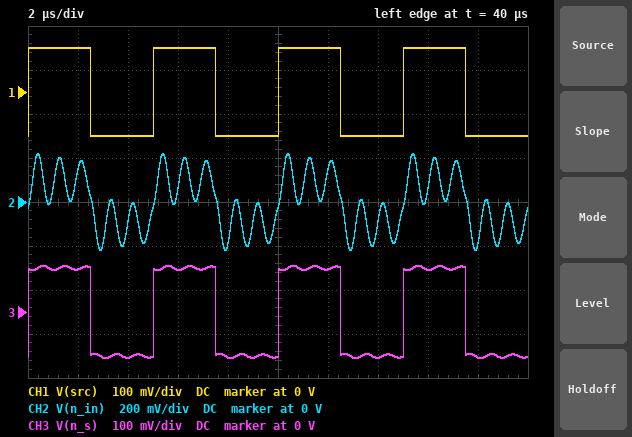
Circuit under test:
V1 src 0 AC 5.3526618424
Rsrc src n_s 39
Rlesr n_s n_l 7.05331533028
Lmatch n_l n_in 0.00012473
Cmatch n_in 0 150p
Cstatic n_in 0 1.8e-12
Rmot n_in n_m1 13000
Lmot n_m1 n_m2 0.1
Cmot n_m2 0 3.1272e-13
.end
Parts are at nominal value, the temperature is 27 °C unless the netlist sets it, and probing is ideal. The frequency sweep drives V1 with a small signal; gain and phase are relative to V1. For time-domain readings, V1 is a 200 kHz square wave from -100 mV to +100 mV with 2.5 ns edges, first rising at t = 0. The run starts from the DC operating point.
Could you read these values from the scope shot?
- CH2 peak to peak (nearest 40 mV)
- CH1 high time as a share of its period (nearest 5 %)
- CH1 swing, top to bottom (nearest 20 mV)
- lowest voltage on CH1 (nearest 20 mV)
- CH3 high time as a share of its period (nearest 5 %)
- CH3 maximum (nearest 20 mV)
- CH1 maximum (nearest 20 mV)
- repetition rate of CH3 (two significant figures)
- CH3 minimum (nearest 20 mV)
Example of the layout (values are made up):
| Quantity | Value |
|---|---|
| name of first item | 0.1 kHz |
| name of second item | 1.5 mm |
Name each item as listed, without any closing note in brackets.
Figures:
| Quantity | Value |
|---|---|
| CH2 peak to peak | 440 mV |
| CH1 high time as a share of its period | 50 % |
| CH1 swing, top to bottom | 200 mV |
| lowest voltage on CH1 | -100 mV |
| CH3 high time as a share of its period | 50 % |
| CH3 maximum | 100 mV |
| CH1 maximum | 100 mV |
| repetition rate of CH3 | 200 kHz |
| CH3 minimum | -100 mV |
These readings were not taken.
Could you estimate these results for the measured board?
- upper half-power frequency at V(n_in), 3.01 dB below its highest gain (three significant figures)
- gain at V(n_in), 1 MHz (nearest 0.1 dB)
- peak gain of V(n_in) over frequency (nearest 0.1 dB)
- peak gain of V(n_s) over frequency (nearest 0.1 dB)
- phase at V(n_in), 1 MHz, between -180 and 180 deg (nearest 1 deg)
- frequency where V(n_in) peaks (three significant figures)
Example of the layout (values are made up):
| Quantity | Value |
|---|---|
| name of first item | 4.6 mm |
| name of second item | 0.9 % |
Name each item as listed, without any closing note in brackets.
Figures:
| Quantity | Value |
|---|---|
| upper half-power frequency at V(n_in), 3.01 dB below its highest gain | 1.19 MHz |
| gain at V(n_in), 1 MHz | 11.6 dB |
| peak gain of V(n_in) over frequency | 25.9 dB |
| peak gain of V(n_s) over frequency | 0 dB |
| phase at V(n_in), 1 MHz, between -180 and 180 deg | -10 deg |
| frequency where V(n_in) peaks | 1.16 MHz |
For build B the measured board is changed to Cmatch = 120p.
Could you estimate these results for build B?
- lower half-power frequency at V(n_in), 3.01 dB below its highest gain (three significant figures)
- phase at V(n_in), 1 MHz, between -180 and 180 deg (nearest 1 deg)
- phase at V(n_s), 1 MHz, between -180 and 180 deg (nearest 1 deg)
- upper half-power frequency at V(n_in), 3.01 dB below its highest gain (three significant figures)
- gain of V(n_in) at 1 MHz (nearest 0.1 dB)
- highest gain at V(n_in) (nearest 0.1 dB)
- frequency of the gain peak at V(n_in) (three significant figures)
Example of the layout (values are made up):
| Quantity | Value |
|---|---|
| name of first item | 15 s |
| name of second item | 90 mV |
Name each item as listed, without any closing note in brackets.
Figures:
| Quantity | Value |
|---|---|
| lower half-power frequency at V(n_in), 3.01 dB below its highest gain | 1.26 MHz |
| phase at V(n_in), 1 MHz, between -180 and 180 deg | -5 deg |
| phase at V(n_s), 1 MHz, between -180 and 180 deg | -4 deg |
| upper half-power frequency at V(n_in), 3.01 dB below its highest gain | 1.32 MHz |
| gain of V(n_in) at 1 MHz | 7.8 dB |
| highest gain at V(n_in) | 26.8 dB |
| frequency of the gain peak at V(n_in) | 1.29 MHz |
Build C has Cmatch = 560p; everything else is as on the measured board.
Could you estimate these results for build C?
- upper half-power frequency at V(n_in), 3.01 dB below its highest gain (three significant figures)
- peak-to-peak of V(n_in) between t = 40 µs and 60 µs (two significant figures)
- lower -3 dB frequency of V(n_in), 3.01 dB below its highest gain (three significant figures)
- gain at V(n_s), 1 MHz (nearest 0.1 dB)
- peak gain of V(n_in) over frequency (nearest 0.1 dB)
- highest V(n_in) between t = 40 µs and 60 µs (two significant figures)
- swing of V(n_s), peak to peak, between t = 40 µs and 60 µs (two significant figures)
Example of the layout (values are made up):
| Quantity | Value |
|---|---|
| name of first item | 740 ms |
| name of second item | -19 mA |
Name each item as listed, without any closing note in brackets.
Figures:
| Quantity | Value |
|---|---|
| upper half-power frequency at V(n_in), 3.01 dB below its highest gain | 628 kHz |
| peak-to-peak of V(n_in) between t = 40 µs and 60 µs | 1.1 V |
| lower -3 dB frequency of V(n_in), 3.01 dB below its highest gain | 569 kHz |
| gain at V(n_s), 1 MHz | 0 dB |
| peak gain of V(n_in) over frequency | 20.2 dB |
| highest V(n_in) between t = 40 µs and 60 µs | 560 mV |
| swing of V(n_s), peak to peak, between t = 40 µs and 60 µs | 270 mV |
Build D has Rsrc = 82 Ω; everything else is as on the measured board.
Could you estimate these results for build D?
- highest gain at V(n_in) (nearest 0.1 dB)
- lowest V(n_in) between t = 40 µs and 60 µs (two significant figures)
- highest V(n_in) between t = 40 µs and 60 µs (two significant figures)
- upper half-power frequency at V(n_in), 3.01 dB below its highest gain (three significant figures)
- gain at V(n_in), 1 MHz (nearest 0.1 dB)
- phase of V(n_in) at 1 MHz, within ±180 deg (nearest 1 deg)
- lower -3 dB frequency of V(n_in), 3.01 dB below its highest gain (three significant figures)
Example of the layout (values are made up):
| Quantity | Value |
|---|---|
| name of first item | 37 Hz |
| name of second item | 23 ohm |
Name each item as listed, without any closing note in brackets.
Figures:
| Quantity | Value |
|---|---|
| highest gain at V(n_in) | 20.2 dB |
| lowest V(n_in) between t = 40 µs and 60 µs | -230 mV |
| highest V(n_in) between t = 40 µs and 60 µs | 230 mV |
| upper half-power frequency at V(n_in), 3.01 dB below its highest gain | 1.21 MHz |
| gain at V(n_in), 1 MHz | 11.3 dB |
| phase of V(n_in) at 1 MHz, within ±180 deg | -18 deg |
| lower -3 dB frequency of V(n_in), 3.01 dB below its highest gain | 1.10 MHz |
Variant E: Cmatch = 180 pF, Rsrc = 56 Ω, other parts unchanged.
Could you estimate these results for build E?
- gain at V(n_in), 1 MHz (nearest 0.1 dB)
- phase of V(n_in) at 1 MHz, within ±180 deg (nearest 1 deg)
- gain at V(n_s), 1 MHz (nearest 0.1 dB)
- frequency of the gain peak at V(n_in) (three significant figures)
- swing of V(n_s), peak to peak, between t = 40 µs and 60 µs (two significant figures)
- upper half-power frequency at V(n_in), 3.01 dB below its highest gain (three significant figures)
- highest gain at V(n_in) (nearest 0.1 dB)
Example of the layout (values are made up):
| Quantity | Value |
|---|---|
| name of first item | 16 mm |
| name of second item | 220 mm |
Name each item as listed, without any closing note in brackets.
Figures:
| Quantity | Value |
|---|---|
| gain at V(n_in), 1 MHz | 17.5 dB |
| phase of V(n_in) at 1 MHz, within ±180 deg | -33 deg |
| gain at V(n_s), 1 MHz | -1.5 dB |
| frequency of the gain peak at V(n_in) | 1.06 MHz |
| swing of V(n_s), peak to peak, between t = 40 µs and 60 µs | 230 mV |
| upper half-power frequency at V(n_in), 3.01 dB below its highest gain | 1.10 MHz |
| highest gain at V(n_in) | 22.4 dB |
